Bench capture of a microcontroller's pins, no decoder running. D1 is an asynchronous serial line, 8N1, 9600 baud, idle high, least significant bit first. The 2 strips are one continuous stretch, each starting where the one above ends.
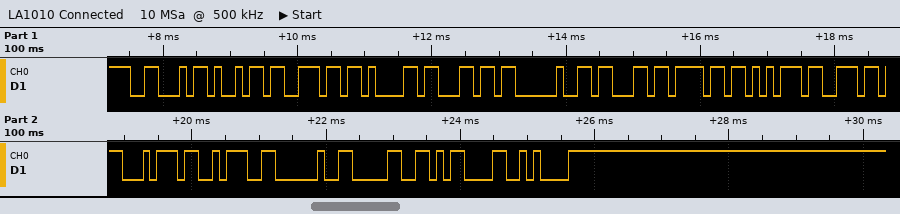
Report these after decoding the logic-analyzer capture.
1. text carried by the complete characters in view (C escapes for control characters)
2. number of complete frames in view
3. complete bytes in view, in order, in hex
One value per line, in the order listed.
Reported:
"Final count: 0\r\n"
16
46 69 6E 61 6C 20 63 6F 75 6E 74 3A 20 30 0D 0A
